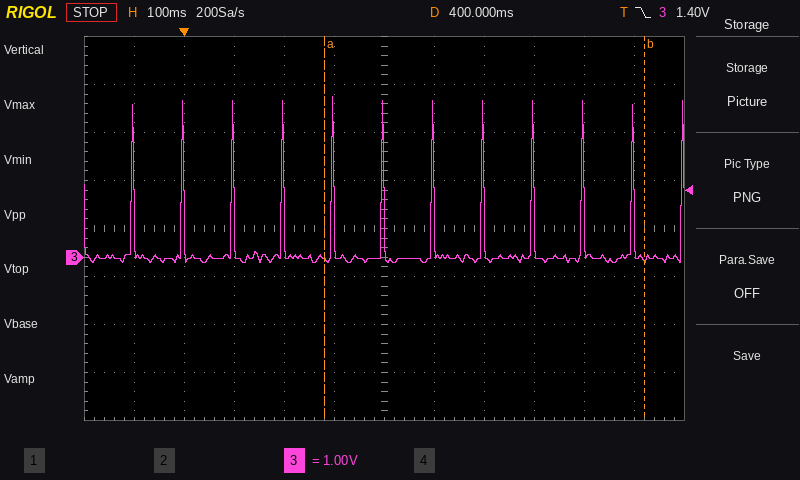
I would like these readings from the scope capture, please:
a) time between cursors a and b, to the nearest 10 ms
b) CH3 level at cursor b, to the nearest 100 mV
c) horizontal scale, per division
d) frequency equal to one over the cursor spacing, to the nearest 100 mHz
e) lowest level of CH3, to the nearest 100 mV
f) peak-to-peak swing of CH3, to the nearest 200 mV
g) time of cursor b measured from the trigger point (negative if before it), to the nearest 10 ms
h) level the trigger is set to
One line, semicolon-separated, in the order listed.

640 ms; 0.0 V; 100 ms; 1.6 Hz; -100 mV; 3.4 V; +920 ms; 1.40 V
